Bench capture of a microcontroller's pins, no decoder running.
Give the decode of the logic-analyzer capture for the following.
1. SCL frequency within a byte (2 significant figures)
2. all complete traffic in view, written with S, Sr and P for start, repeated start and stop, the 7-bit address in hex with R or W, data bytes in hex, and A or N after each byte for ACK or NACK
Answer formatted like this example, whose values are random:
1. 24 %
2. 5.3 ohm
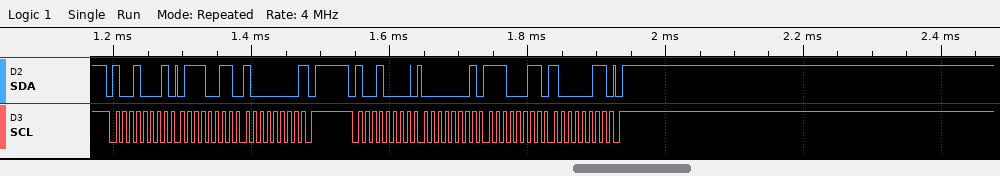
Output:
1. 100 kHz
2. S 48R A 73 A 80 N P S 48W A 01 A E3 A 83 A P
